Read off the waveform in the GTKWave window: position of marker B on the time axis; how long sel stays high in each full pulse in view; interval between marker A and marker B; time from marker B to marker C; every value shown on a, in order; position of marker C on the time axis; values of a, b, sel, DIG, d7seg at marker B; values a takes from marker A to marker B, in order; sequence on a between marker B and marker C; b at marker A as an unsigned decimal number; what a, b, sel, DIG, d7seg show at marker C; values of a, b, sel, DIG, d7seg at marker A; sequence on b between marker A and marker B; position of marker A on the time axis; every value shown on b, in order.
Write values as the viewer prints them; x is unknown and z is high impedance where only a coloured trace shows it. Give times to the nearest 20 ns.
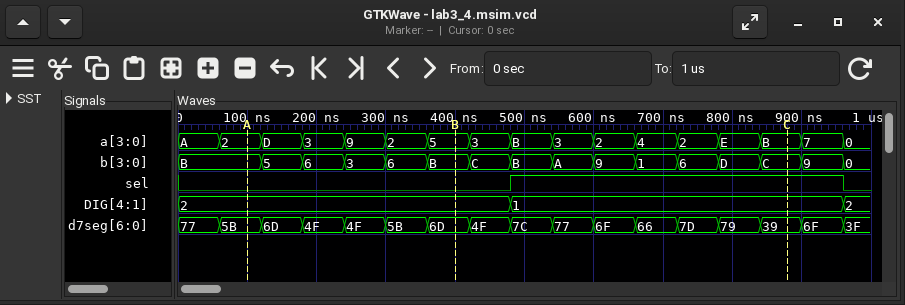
400 ns
480 ns
300 ns
480 ns
A, 2, D, 3, 9, 2, 5, 3, B, 3, 2, 4, 2, E, B, 7, 0
880 ns
a=5, b=B, sel=0, DIG=2, d7seg=6D
2, D, 3, 9, 2, 5
5, 3, B, 3, 2, 4, 2, E, B
11
a=B, b=C, sel=1, DIG=1, d7seg=39
a=2, b=B, sel=0, DIG=2, d7seg=5B
B, 5, 6, 3, 6, B
100 ns
B, 5, 6, 3, 6, B, C, B, A, 9, 1, 6, D, C, 9, 0
